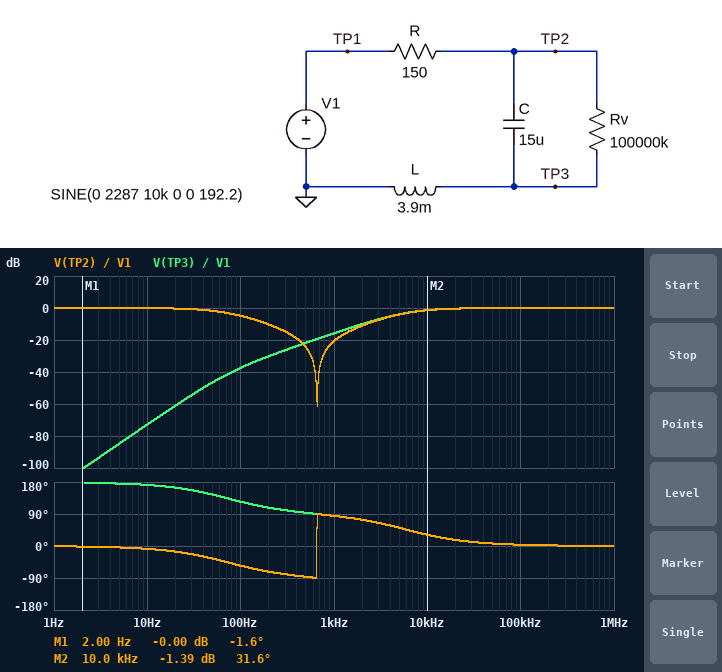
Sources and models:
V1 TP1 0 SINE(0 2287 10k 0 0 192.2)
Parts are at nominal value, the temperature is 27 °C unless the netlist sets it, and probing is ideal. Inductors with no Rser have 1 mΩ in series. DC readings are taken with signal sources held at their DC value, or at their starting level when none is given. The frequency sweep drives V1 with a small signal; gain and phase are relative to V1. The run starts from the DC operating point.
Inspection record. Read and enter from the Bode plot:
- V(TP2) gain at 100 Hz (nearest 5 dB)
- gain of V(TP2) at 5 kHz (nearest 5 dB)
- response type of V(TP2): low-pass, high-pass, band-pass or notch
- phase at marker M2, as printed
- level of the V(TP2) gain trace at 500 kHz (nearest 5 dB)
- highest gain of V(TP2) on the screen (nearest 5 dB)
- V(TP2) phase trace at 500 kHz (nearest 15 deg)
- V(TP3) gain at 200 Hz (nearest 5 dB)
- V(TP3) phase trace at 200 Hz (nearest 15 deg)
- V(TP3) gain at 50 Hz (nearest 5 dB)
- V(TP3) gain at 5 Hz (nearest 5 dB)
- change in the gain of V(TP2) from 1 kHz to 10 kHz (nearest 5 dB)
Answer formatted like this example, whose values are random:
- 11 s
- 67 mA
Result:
- -5 dB
- -5 dB
- notch
- 31.6 deg
- 0 dB
- 0 dB
- 0 deg
- -30 dB
- 105 deg
- -45 dB
- -85 dB
- 20 dB
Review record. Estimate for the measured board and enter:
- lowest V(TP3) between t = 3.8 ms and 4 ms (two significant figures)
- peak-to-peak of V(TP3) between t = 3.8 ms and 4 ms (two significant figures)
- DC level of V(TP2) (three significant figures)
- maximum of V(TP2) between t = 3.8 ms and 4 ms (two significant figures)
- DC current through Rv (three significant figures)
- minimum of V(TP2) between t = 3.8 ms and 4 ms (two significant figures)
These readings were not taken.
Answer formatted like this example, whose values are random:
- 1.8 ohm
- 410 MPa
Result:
- -2.0 kV
- 3.9 kV
- -483 V
- 1.9 kV
- 4.83 µA
- -2.0 kV
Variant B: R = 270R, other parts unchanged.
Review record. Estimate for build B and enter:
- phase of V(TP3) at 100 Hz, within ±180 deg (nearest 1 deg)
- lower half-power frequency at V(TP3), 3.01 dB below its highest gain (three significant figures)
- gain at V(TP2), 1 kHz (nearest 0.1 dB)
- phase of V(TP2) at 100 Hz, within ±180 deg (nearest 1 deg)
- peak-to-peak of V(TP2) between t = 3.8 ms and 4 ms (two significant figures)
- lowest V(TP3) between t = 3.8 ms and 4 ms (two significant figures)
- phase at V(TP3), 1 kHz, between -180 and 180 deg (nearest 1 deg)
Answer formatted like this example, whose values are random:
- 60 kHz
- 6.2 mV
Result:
- 111 deg
- 11.0 kHz
- -25.8 dB
- -69 deg
- 3.1 kV
- -1.5 kV
- 87 deg
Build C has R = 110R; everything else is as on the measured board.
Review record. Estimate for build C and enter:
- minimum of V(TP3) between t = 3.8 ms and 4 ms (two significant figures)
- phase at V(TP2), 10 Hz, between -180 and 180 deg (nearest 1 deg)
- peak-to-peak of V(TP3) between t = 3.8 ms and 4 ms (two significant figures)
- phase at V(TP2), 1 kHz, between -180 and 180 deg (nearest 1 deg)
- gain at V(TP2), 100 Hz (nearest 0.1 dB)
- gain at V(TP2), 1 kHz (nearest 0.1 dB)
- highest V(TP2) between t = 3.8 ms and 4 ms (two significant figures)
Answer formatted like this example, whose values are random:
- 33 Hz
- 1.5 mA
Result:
- -2.1 kV
- -6 deg
- 4.2 kV
- 83 deg
- -3.3 dB
- -18.0 dB
- 2.0 kV
